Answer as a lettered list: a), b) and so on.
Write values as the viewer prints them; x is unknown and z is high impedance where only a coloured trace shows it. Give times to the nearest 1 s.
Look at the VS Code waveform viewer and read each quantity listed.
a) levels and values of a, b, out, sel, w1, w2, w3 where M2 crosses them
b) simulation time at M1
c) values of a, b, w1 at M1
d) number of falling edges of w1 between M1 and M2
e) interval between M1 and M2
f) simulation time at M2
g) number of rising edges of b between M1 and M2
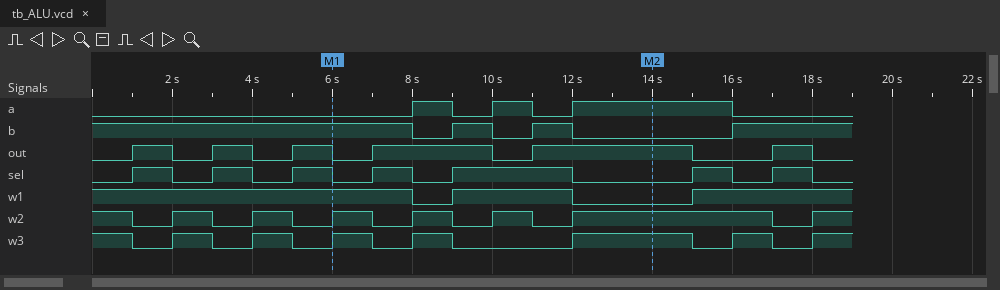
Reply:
a) a=1, b=0, out=1, sel=0, w1=0, w2=1, w3=1
b) 6 s
c) a=0, b=1, w1=1
d) 2
e) 8 s
f) 14 s
g) 2
